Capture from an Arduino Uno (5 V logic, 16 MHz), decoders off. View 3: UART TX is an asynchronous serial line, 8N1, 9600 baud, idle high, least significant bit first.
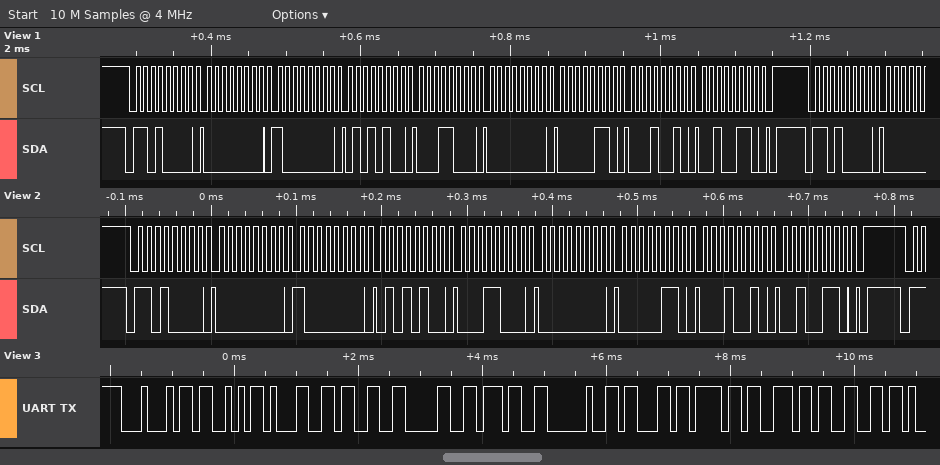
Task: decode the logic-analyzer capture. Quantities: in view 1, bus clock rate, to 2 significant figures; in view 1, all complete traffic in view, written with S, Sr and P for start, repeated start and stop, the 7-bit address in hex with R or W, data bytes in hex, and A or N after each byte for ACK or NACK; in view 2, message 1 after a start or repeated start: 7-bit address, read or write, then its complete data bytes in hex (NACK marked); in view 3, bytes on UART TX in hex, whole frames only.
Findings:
100 kHz
S 68W A 00 A 80 A 54 A 18 A 00 A 06 A 12 A 26 A P S 68W A
0x68 write: 00 80 54 18 00 06 12 26
44 53 31 33 30 37 20 63 6F 6E 66
